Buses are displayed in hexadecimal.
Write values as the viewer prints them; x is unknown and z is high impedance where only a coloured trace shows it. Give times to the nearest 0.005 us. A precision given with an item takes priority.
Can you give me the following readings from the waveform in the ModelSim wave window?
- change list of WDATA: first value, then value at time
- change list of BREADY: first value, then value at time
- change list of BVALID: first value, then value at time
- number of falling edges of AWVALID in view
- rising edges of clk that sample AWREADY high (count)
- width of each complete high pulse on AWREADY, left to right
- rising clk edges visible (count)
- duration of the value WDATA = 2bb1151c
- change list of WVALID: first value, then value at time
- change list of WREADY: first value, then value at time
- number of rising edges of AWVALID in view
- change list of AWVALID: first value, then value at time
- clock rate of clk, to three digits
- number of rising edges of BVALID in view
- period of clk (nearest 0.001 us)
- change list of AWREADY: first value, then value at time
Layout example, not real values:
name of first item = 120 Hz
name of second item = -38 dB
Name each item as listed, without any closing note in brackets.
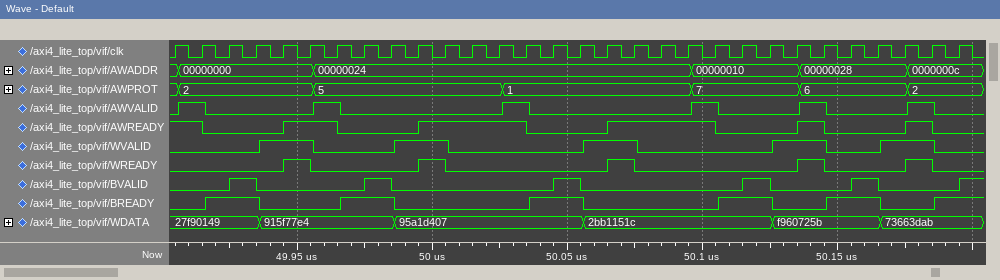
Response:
change list of WDATA: first value, then value at time = 27f90149, 915f77e4 at 49.935 us, 95a1d407 at 49.985 us, 2bb1151c at 50.055 us, f960725b at 50.125 us, 73663dab at 50.165 us
change list of BREADY: first value, then value at time = 0, 1 at 49.915 us, 0 at 49.935 us, 1 at 49.965 us, 0 at 49.985 us, 1 at 50.035 us, 0 at 50.055 us, 1 at 50.105 us, 0 at 50.125 us, 1 at 50.145 us, 0 at 50.165 us, 1 at 50.185 us
change list of BVALID: first value, then value at time = 0, 1 at 49.925 us, 0 at 49.935 us, 1 at 49.975 us, 0 at 49.985 us, 1 at 50.045 us, 0 at 50.055 us, 1 at 50.115 us, 0 at 50.125 us, 1 at 50.155 us, 0 at 50.165 us, 1 at 50.195 us
number of falling edges of AWVALID in view = 6
rising edges of clk that sample AWREADY high = 14
width of each complete high pulse on AWREADY, left to right = 0.02 us, 0.04 us, 0.04 us, 0.01 us, 0.01 us
rising clk edges visible = 30
duration of the value WDATA = 2bb1151c = 0.07 us
change list of WVALID: first value, then value at time = 0, 1 at 49.935 us, 0 at 49.955 us, 1 at 49.985 us, 0 at 50.005 us, 1 at 50.055 us, 0 at 50.075 us, 1 at 50.125 us, 0 at 50.145 us, 1 at 50.165 us, 0 at 50.185 us
change list of WREADY: first value, then value at time = 0, 1 at 49.945 us, 0 at 49.955 us, 1 at 49.995 us, 0 at 50.005 us, 1 at 50.065 us, 0 at 50.075 us, 1 at 50.135 us, 0 at 50.145 us, 1 at 50.175 us, 0 at 50.185 us
number of rising edges of AWVALID in view = 6
change list of AWVALID: first value, then value at time = 0, 1 at 49.905 us, 0 at 49.915 us, 1 at 49.955 us, 0 at 49.965 us, 1 at 50.025 us, 0 at 50.035 us, 1 at 50.095 us, 0 at 50.105 us, 1 at 50.135 us, 0 at 50.145 us, 1 at 50.175 us, 0 at 50.185 us
clock rate of clk, to three digits = 100 MHz
number of rising edges of BVALID in view = 6
period of clk = 0.01 us
change list of AWREADY: first value, then value at time = 1, 0 at 49.915 us, 1 at 49.945 us, 0 at 49.965 us, 1 at 49.995 us, 0 at 50.035 us, 1 at 50.065 us, 0 at 50.105 us, 1 at 50.135 us, 0 at 50.145 us, 1 at 50.175 us, 0 at 50.185 us
